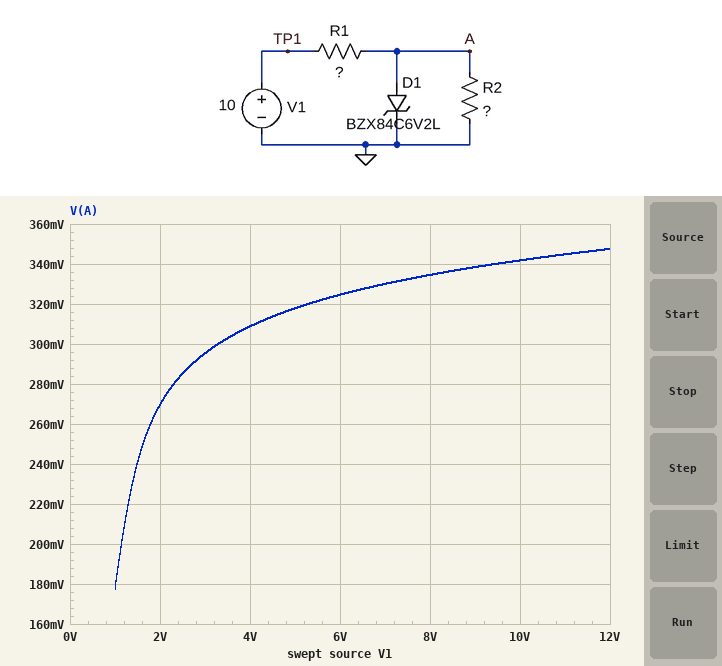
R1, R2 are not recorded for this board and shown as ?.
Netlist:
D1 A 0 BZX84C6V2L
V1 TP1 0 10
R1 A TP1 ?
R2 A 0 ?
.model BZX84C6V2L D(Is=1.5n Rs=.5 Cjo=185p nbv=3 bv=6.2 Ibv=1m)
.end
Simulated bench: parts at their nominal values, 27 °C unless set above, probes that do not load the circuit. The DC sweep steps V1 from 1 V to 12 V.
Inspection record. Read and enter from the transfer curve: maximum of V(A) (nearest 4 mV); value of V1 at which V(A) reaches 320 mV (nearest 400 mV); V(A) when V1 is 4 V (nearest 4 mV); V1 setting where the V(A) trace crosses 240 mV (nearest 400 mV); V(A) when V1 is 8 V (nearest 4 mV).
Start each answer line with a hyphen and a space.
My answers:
- 348 mV
- 5.2 V
- 308 mV
- 1.6 V
- 336 mV
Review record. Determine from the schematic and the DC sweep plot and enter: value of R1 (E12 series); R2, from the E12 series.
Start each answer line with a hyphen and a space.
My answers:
- 10 kΩ
- 2.2 kΩ
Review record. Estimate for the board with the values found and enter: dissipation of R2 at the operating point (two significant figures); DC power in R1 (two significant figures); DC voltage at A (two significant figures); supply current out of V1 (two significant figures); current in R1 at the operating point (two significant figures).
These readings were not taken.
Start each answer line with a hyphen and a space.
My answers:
- 53 µW
- 9.3 mW
- 340 mV
- 970 µA
- 970 µA
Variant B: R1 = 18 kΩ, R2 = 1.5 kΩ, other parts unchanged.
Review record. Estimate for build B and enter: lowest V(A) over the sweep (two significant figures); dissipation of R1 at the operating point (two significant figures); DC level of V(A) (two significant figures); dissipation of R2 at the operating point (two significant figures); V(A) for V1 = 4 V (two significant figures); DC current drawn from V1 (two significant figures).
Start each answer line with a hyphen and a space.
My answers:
- 77 mV
- 5.2 mW
- 320 mV
- 67 µW
- 260 mV
- 540 µA
